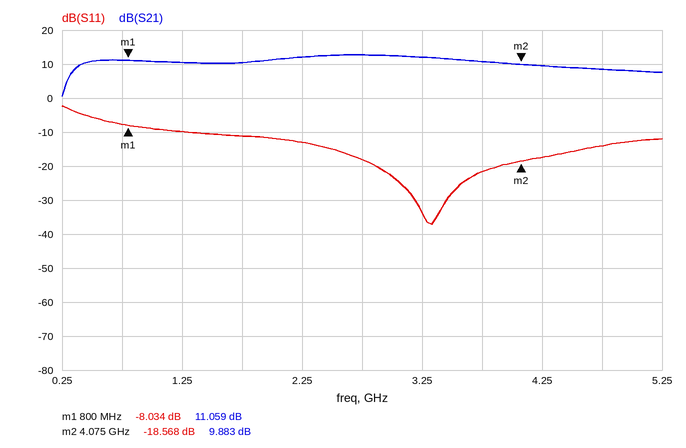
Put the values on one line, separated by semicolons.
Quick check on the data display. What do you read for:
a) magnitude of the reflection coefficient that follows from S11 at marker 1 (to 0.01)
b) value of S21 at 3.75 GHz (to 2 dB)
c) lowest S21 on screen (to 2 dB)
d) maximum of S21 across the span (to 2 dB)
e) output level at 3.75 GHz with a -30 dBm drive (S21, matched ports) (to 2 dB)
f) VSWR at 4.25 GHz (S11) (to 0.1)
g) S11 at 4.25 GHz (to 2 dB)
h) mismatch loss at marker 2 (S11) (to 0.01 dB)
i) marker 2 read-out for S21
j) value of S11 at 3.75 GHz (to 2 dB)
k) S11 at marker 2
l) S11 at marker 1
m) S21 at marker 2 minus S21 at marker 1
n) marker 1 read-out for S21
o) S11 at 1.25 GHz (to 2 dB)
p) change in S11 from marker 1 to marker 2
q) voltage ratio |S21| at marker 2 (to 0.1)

0.40; 10 dB; 0 dB; 12 dB; -20 dBm; 1.3; -18 dB; 0.06 dB; 9.883 dB; -22 dB; -18.568 dB; -8.034 dB; -1.176 dB; 11.059 dB; -10 dB; -10.534 dB; 3.1
